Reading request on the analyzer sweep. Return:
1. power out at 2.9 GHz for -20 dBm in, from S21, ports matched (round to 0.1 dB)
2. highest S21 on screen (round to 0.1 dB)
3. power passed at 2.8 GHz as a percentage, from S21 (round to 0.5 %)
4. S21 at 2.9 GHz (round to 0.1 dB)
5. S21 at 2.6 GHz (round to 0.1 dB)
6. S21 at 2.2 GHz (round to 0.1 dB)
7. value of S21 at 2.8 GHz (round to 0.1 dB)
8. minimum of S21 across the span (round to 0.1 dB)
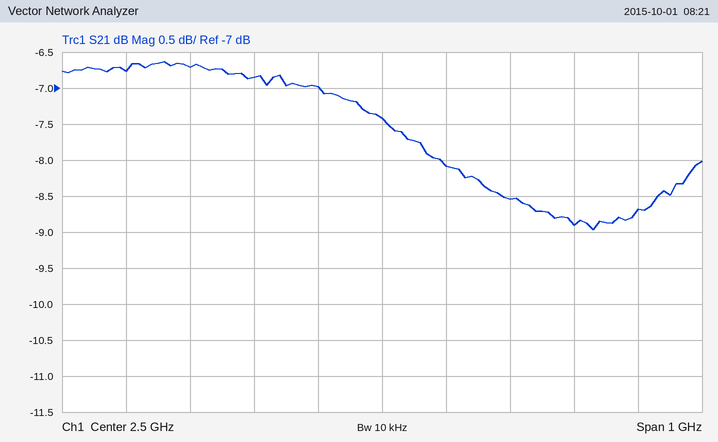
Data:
-28.7 dBm
-6.6 dB
13.0 %
-8.7 dB
-8.1 dB
-6.7 dB
-8.9 dB
-9.0 dB
